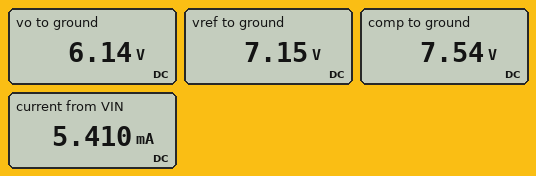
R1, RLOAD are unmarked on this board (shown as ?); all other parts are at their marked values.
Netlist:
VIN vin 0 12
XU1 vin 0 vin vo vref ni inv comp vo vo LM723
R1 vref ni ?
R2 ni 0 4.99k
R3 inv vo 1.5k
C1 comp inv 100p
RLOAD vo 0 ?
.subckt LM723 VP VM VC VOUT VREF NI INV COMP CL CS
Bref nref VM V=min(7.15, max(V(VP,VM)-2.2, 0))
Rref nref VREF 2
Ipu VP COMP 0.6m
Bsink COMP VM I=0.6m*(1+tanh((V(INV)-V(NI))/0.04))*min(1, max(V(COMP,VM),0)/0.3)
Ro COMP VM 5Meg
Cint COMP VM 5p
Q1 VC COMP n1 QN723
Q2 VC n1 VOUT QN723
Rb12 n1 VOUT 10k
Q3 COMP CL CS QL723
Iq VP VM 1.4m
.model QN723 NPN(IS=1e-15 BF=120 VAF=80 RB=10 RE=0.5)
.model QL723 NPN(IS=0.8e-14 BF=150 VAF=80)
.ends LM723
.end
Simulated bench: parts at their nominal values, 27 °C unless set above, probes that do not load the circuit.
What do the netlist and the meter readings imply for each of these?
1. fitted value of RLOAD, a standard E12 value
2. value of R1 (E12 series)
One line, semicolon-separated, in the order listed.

1.8 kΩ; 820 Ω
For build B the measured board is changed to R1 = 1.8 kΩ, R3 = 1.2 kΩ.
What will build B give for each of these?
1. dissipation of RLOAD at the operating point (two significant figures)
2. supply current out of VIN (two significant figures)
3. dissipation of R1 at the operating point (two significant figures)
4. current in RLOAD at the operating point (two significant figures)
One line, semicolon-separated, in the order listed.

15 mW; 4.9 mA; 2.0 mW; 2.9 mA
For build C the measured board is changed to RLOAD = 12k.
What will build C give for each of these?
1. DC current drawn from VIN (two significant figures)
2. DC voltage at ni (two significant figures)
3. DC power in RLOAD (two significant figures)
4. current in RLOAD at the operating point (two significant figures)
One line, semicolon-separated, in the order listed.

2.5 mA; 6.1 V; 3.1 mW; 510 µA
